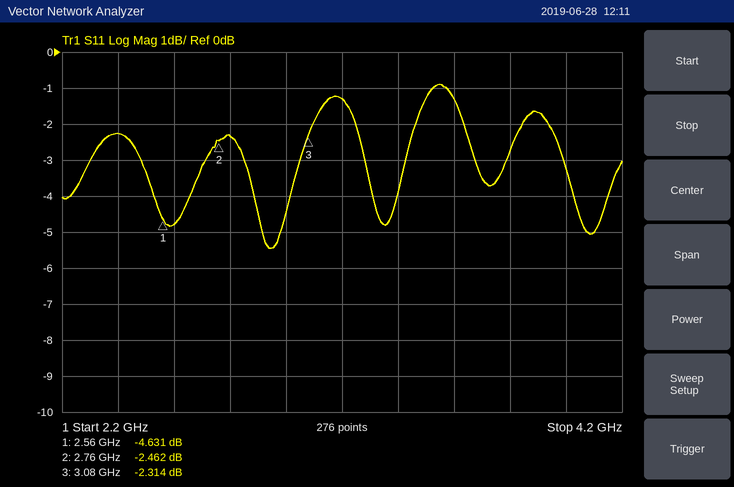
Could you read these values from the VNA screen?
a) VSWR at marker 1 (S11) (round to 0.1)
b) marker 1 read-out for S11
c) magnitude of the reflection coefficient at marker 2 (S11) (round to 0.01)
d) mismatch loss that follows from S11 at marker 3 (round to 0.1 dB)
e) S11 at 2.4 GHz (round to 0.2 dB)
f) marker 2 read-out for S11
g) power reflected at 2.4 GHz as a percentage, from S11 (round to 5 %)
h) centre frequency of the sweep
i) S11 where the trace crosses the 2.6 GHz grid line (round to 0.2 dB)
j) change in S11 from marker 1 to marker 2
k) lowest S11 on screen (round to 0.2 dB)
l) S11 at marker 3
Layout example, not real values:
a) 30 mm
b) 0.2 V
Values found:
a) 3.8
b) -4.631 dB
c) 0.75
d) 3.8 dB
e) -2.2 dB
f) -2.462 dB
g) 60 %
h) 3.2 GHz
i) -4.8 dB
j) 2.169 dB
k) -5.4 dB
l) -2.314 dB
